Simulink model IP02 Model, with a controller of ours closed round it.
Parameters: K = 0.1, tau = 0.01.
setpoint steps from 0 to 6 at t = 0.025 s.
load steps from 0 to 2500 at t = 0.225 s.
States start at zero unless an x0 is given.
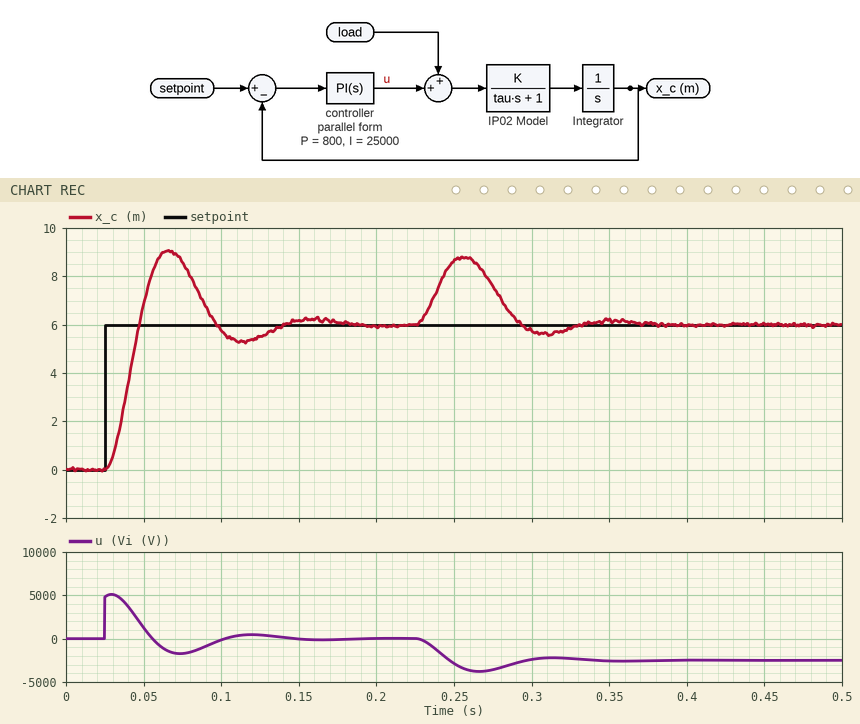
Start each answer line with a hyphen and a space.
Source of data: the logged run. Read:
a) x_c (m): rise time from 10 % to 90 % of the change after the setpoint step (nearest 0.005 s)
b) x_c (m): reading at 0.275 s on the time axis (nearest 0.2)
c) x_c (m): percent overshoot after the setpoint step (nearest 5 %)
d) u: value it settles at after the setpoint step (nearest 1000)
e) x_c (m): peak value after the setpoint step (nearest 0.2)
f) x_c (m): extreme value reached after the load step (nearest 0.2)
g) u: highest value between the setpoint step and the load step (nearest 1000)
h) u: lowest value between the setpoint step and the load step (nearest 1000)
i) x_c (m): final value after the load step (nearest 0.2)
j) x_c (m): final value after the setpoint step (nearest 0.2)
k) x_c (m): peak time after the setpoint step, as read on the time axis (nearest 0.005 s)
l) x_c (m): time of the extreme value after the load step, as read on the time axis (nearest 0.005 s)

- 0.015 s
- 7.6
- 50 %
- 0
- 9.0
- 8.8
- 5000
- -2000
- 6.0
- 6.0
- 0.065 s
- 0.255 s
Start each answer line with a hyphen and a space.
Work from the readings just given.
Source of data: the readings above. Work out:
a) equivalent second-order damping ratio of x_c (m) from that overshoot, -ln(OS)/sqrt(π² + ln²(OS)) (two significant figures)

- 0.22
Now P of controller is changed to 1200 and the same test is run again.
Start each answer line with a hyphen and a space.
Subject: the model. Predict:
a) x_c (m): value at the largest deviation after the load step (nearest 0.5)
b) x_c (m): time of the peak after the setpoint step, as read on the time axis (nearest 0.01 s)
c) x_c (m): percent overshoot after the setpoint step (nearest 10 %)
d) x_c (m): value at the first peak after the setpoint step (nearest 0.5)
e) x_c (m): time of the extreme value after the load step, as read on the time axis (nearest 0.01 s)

- 8.0
- 0.06 s
- 40 %
- 8.5
- 0.25 s
